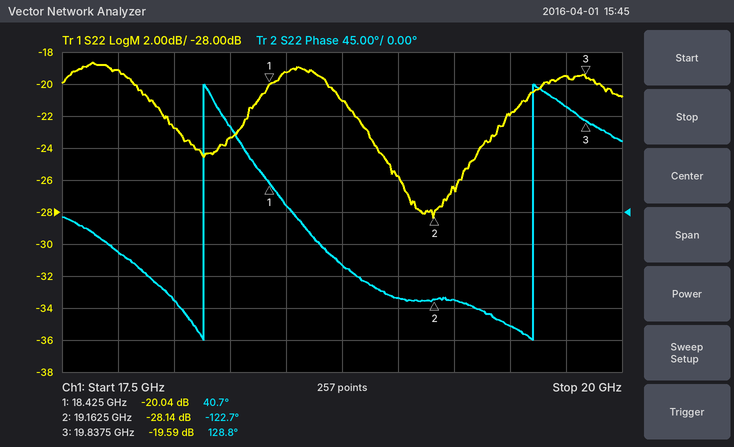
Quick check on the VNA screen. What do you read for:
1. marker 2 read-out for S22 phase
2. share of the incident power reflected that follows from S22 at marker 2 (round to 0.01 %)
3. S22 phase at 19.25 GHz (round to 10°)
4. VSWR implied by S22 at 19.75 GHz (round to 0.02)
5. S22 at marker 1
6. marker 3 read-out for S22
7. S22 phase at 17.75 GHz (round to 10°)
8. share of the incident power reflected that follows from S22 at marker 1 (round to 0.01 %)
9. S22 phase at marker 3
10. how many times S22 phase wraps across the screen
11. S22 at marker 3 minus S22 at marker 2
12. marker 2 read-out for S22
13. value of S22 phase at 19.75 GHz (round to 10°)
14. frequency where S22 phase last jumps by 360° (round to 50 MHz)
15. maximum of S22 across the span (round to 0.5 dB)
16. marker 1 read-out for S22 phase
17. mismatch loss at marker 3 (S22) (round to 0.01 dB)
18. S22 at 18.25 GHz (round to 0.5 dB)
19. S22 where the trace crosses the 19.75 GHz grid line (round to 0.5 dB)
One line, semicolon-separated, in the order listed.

-122.7°; 0.15 %; -120°; 1.24; -20.04 dB; -19.59 dB; -60°; 0.99 %; 128.8°; 2; 8.55 dB; -28.14 dB; 150°; 19.60 GHz; -18.5 dB; 40.7°; 0.05 dB; -23.5 dB; -19.5 dB
